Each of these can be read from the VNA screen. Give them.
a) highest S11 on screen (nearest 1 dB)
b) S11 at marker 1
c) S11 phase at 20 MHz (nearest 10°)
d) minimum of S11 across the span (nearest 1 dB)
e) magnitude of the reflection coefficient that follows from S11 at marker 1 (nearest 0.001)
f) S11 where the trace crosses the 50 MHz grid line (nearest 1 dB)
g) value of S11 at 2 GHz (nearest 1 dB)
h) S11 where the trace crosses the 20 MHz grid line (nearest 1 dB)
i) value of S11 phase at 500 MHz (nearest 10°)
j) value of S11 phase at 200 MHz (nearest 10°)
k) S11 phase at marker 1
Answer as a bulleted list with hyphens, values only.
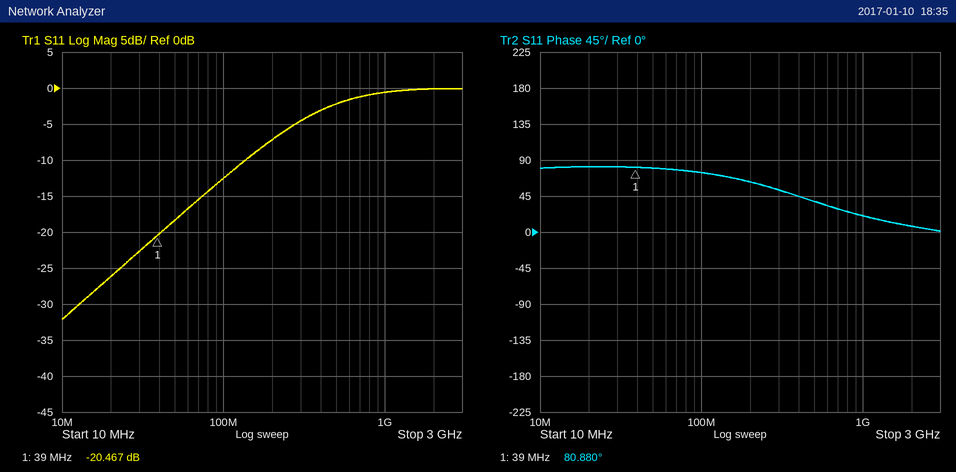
- 0 dB
- -20.467 dB
- 80°
- -32 dB
- 0.095
- -18 dB
- 0 dB
- -26 dB
- 40°
- 60°
- 80.880°
